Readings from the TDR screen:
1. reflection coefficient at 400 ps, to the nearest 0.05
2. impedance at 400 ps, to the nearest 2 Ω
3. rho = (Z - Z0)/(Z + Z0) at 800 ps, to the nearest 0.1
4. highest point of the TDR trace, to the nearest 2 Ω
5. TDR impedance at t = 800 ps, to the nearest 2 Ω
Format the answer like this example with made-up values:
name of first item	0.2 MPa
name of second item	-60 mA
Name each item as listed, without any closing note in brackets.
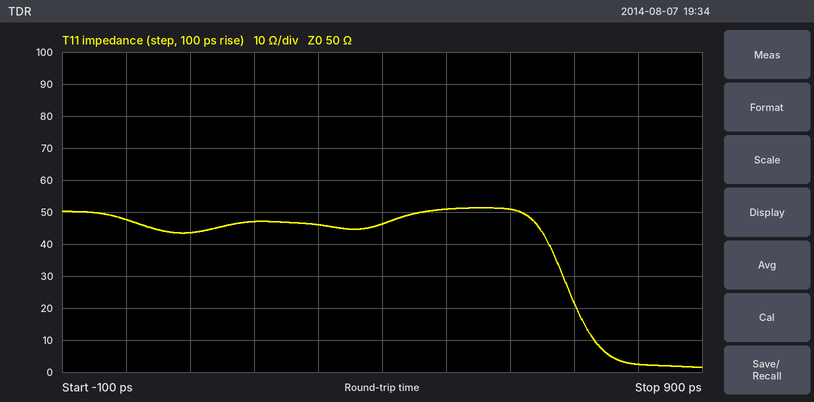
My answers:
reflection coefficient at 400 ps, to the nearest 0.05	-0.05
impedance at 400 ps, to the nearest 2 Ω	46 Ω
rho = (Z - Z0)/(Z + Z0) at 800 ps, to the nearest 0.1	-0.9
highest point of the TDR trace, to the nearest 2 Ω	52 Ω
TDR impedance at t = 800 ps, to the nearest 2 Ω	2 Ω
